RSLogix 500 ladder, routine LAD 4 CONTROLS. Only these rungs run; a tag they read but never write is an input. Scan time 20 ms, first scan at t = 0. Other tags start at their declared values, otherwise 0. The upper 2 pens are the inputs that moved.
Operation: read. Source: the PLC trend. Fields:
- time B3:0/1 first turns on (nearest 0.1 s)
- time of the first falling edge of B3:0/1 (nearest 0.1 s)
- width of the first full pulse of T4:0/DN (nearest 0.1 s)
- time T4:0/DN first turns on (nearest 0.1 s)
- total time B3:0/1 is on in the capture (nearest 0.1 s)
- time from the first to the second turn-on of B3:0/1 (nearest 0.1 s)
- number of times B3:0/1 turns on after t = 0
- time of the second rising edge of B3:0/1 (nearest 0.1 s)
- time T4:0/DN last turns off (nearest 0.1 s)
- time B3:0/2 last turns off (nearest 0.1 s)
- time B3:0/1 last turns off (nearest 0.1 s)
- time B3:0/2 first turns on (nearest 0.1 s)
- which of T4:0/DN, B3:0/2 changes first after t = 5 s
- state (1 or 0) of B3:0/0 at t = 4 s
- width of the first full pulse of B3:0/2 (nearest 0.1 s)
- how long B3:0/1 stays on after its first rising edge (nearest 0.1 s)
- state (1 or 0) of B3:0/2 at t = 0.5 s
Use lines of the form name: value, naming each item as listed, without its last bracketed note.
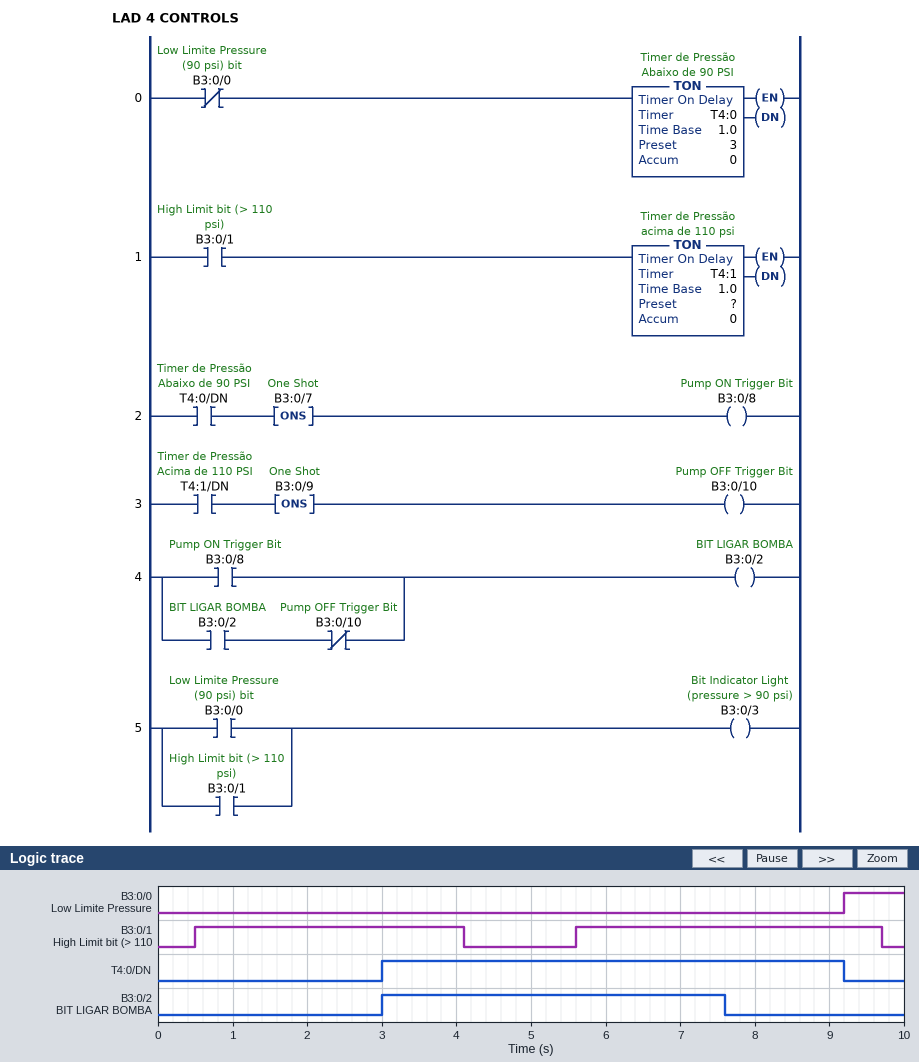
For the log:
time B3:0/1 first turns on: 0.5 s
time of the first falling edge of B3:0/1: 4.1 s
width of the first full pulse of T4:0/DN: 6.2 s
time T4:0/DN first turns on: 3.0 s
total time B3:0/1 is on in the capture: 7.7 s
time from the first to the second turn-on of B3:0/1: 5.1 s
number of times B3:0/1 turns on after t = 0: 2
time of the second rising edge of B3:0/1: 5.6 s
time T4:0/DN last turns off: 9.2 s
time B3:0/2 last turns off: 7.6 s
time B3:0/1 last turns off: 9.7 s
time B3:0/2 first turns on: 3.0 s
which of T4:0/DN, B3:0/2 changes first after t = 5 s: B3:0/2
state (1 or 0) of B3:0/0 at t = 4 s: 0
width of the first full pulse of B3:0/2: 4.6 s
how long B3:0/1 stays on after its first rising edge: 3.6 s
state (1 or 0) of B3:0/2 at t = 0.5 s: 0
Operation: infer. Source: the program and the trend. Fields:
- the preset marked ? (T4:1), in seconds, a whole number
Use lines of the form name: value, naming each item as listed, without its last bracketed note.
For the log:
the preset marked ? (T4:1), in seconds, a whole number: 2 s
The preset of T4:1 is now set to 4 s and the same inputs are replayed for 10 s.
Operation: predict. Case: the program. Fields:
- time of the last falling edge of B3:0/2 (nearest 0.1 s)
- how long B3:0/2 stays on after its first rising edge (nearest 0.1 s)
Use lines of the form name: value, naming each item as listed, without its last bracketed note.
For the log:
time of the last falling edge of B3:0/2: 9.6 s
how long B3:0/2 stays on after its first rising edge: 6.6 s
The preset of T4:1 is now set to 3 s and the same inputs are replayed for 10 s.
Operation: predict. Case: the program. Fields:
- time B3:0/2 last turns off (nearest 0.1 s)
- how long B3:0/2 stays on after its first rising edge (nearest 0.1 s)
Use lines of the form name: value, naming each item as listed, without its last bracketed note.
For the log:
time B3:0/2 last turns off: 3.5 s
how long B3:0/2 stays on after its first rising edge: 0.5 s
